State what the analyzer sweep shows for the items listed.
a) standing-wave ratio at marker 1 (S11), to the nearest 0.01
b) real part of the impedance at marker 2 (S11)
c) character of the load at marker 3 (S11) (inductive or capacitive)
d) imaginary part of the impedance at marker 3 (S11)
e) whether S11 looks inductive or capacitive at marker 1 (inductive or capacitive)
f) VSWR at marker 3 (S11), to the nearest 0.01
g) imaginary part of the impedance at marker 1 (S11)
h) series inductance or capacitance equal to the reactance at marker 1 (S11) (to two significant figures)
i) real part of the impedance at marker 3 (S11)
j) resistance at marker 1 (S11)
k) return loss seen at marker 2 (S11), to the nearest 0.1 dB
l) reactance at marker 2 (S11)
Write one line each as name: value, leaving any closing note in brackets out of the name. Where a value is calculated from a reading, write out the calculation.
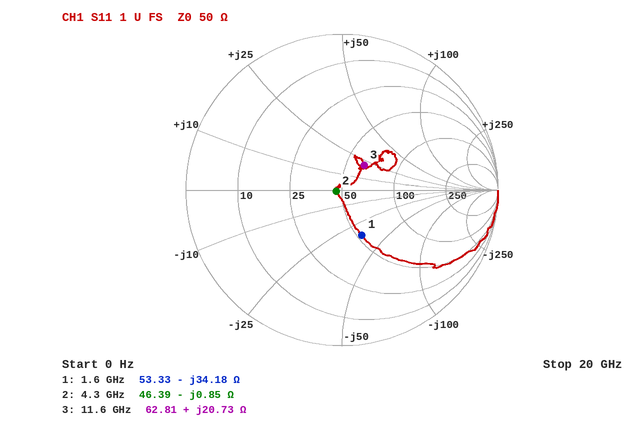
standing-wave ratio at marker 1 (S11), to the nearest 0.01: 1.92
real part of the impedance at marker 2: 46.39 Ω
character of the load at marker 3 (S11): inductive
imaginary part of the impedance at marker 3: +20.73 Ω
whether S11 looks inductive or capacitive at marker 1: capacitive
VSWR at marker 3 (S11), to the nearest 0.01: 1.54
imaginary part of the impedance at marker 1: -34.18 Ω
series inductance or capacitance equal to the reactance at marker 1 (S11): C = 1/(2π × 1.6 GHz × 34.18 Ω) ≈ 2.9 pF
real part of the impedance at marker 3: 62.81 Ω
resistance at marker 1: 53.33 Ω
return loss seen at marker 2 (S11), to the nearest 0.1 dB: 28.3 dB
reactance at marker 2: -0.85 Ω
